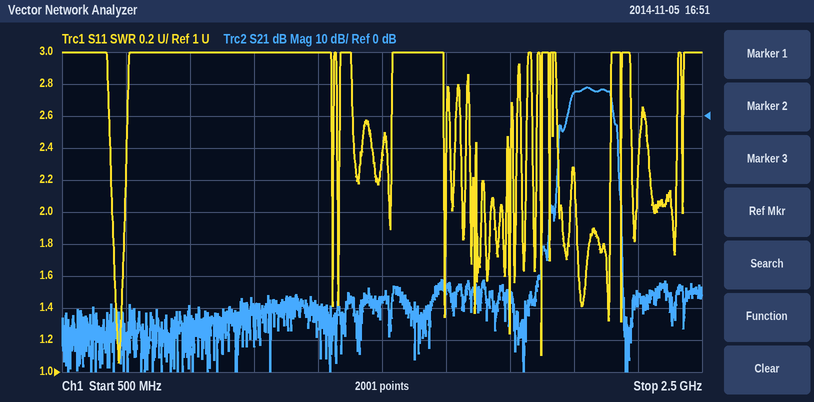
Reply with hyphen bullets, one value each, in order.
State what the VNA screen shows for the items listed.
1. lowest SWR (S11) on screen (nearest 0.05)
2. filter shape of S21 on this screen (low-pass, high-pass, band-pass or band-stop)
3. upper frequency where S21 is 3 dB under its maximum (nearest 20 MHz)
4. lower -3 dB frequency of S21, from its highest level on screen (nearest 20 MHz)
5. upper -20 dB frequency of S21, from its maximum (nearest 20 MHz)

- 1.05
- band-pass
- 2.22 GHz
- 2.10 GHz
- 2.24 GHz
